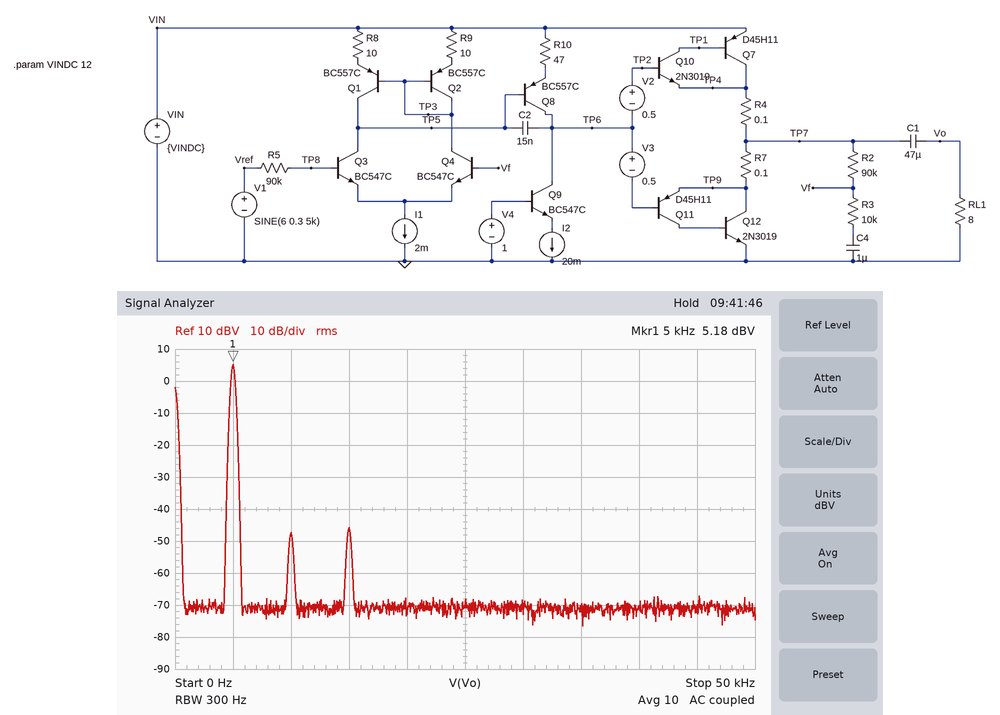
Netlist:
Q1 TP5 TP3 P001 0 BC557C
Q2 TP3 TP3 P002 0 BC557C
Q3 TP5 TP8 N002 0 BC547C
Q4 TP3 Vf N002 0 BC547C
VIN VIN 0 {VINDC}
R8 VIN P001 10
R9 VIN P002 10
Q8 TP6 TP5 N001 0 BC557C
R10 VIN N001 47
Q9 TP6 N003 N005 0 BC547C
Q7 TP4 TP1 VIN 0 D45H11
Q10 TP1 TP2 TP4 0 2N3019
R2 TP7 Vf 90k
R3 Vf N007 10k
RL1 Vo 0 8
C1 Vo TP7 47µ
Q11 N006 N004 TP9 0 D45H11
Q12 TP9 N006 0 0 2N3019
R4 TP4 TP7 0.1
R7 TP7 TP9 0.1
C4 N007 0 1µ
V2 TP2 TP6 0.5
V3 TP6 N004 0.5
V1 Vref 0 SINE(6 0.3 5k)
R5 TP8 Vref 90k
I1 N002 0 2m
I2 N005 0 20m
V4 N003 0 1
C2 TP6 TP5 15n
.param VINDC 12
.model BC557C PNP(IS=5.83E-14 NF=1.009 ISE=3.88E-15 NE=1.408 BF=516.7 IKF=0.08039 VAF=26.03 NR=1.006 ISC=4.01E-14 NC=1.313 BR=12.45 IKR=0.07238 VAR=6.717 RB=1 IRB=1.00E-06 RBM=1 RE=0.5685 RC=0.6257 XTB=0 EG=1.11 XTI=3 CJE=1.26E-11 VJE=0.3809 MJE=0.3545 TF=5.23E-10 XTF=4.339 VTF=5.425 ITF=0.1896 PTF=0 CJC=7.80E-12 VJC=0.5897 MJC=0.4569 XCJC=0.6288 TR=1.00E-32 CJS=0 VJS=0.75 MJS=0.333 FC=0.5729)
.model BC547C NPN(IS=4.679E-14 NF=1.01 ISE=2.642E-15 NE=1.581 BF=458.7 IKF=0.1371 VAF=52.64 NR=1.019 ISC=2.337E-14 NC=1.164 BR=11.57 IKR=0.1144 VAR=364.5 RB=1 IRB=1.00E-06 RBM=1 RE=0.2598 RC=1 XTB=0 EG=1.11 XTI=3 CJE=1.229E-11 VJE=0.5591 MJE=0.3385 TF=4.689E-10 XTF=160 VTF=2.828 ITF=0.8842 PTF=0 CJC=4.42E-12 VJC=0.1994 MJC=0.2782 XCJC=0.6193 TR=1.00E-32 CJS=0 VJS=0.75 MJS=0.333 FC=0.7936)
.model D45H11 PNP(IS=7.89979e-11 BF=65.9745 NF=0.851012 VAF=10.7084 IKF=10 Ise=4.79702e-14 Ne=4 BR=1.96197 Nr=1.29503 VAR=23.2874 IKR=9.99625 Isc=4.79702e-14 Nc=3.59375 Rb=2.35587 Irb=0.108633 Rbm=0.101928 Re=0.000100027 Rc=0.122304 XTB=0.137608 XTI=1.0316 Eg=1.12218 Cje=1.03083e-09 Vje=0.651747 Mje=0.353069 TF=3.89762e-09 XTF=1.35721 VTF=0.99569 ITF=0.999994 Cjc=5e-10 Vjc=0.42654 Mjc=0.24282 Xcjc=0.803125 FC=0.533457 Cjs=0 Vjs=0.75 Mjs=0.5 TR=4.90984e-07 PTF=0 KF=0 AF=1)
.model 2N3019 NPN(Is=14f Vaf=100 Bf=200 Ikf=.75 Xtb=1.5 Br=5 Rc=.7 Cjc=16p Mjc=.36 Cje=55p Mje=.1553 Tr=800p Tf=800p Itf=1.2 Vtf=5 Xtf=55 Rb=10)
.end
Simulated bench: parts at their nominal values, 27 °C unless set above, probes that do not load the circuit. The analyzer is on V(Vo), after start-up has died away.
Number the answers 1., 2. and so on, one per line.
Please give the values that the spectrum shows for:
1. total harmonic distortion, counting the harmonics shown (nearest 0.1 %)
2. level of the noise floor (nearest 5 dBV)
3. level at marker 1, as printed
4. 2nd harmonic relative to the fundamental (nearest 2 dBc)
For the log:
1. 0.4 %
2. -70 dBV
3. 5.18 dBV
4. -52 dBc
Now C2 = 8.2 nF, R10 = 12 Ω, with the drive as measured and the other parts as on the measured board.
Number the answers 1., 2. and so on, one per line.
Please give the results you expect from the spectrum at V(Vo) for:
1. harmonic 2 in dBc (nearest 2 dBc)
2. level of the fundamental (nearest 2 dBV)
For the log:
1. -58 dBc
2. 6 dBV
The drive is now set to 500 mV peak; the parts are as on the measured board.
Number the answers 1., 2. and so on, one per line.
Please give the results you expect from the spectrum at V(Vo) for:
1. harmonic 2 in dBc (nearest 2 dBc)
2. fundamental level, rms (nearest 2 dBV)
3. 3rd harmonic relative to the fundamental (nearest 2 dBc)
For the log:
1. -42 dBc
2. 10 dBV
3. -36 dBc
